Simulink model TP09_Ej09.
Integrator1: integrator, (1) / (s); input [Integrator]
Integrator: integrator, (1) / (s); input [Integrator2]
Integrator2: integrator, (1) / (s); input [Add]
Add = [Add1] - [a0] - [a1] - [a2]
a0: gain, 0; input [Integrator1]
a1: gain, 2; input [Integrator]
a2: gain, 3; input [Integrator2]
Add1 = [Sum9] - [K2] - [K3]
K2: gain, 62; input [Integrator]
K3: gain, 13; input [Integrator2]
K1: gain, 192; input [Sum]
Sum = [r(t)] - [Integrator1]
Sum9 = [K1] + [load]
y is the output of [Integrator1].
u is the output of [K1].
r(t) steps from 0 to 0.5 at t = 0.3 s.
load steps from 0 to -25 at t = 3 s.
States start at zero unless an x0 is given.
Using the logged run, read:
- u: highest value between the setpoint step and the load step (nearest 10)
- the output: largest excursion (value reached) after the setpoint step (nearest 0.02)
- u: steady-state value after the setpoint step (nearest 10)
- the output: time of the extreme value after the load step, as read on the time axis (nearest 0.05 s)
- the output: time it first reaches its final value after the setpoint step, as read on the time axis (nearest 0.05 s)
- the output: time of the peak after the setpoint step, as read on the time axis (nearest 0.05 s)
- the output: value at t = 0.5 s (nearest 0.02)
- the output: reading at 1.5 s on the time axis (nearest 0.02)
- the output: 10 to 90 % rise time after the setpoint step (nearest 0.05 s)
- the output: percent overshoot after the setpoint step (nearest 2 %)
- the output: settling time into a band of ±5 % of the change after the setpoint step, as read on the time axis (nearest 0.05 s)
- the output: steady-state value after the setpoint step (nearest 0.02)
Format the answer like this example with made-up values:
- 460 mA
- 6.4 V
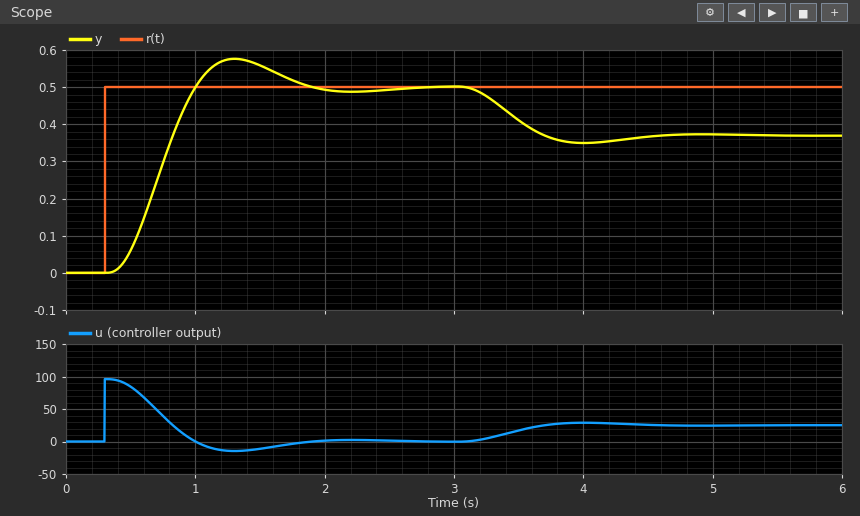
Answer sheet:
- 100
- 0.58
- 0
- 4.00 s
- 1.00 s
- 1.30 s
- 0.06
- 0.56
- 0.45 s
- 16 %
- 1.70 s
- 0.50
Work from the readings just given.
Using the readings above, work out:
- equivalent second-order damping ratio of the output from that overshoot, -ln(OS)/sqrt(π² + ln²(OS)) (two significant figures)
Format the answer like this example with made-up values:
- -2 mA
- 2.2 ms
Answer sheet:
- 0.50
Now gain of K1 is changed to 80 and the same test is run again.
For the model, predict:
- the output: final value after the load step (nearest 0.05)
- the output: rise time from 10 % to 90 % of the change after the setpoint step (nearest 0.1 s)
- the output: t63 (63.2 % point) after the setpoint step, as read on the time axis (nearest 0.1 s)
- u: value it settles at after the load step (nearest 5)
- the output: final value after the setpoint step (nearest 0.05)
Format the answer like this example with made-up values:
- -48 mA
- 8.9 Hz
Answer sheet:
- 0.20
- 1.2 s
- 1.2 s
- 25
- 0.50
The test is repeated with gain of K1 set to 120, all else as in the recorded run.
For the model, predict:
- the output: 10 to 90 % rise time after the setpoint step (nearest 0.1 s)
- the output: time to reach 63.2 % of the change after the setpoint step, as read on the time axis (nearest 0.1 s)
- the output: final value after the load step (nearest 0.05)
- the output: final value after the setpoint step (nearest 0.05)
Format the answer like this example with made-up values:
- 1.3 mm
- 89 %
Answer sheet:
- 0.7 s
- 0.9 s
- 0.30
- 0.50
